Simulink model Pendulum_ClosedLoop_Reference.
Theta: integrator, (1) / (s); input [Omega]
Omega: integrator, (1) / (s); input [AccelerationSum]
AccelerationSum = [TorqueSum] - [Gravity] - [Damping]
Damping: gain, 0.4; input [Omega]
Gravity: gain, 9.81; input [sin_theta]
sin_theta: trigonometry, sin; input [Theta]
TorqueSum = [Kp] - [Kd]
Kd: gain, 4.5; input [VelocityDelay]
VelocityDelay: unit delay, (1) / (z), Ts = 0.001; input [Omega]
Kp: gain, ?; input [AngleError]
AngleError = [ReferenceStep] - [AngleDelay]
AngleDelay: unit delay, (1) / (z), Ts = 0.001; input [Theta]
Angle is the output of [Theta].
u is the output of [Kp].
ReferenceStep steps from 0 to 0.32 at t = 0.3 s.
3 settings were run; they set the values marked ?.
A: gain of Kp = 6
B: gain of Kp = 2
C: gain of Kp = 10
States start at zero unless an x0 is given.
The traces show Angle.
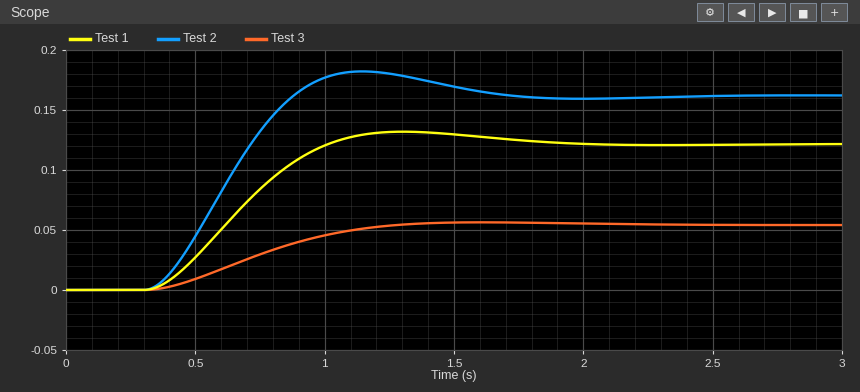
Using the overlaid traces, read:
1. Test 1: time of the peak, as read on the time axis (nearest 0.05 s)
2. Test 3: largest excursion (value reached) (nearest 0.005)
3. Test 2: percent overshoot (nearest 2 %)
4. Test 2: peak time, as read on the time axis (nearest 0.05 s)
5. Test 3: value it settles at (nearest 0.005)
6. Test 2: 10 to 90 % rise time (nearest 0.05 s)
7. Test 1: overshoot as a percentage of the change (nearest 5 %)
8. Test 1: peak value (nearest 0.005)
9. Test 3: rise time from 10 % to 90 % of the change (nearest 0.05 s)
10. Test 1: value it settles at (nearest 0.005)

1.30 s
0.055
12 %
1.15 s
0.055
0.40 s
10 %
0.130
0.65 s
0.120
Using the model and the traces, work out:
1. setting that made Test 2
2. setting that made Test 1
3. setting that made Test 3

C
A
B
